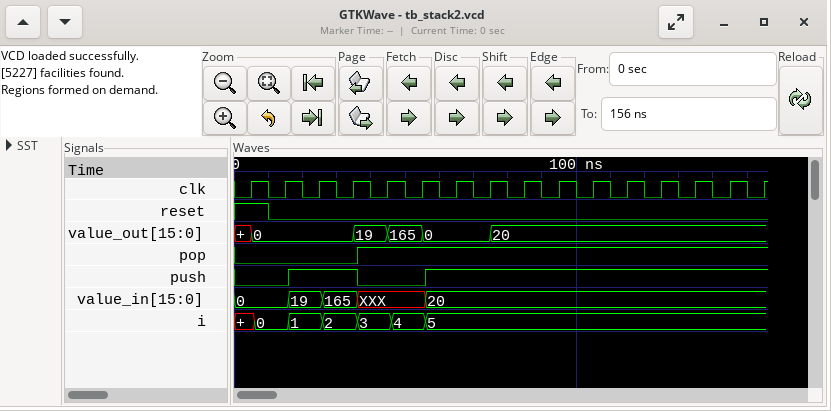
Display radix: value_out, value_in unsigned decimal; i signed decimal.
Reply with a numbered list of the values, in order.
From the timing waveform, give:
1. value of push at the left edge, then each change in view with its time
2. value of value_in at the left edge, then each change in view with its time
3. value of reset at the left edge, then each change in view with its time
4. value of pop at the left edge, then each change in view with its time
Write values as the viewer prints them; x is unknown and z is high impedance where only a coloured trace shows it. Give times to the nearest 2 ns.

1. 0, 1 at 16 ns, 0 at 36 ns, 1 at 56 ns
2. 0, 19 at 16 ns, 165 at 26 ns, XXX at 36 ns, 20 at 56 ns
3. 1, 0 at 10 ns
4. 0, 1 at 36 ns
